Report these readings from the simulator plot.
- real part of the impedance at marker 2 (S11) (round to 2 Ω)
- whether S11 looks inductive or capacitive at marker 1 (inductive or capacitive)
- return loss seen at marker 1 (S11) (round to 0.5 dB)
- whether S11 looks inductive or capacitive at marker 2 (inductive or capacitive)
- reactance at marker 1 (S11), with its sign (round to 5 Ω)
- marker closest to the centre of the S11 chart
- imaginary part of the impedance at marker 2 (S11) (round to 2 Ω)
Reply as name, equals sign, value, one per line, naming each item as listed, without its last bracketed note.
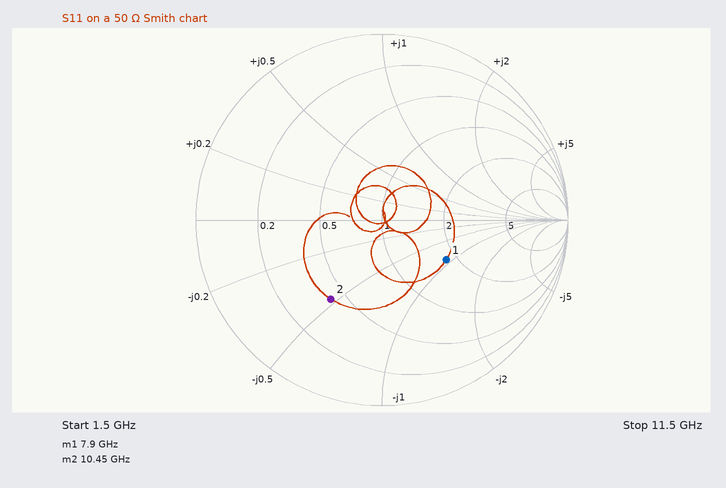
real part of the impedance at marker 2 (S11) = 20 Ω
whether S11 looks inductive or capacitive at marker 1 = capacitive
return loss seen at marker 1 (S11) = 8.0 dB
whether S11 looks inductive or capacitive at marker 2 = capacitive
reactance at marker 1 (S11), with its sign = -45 Ω
marker closest to the centre of the S11 chart = marker 1
imaginary part of the impedance at marker 2 (S11) = -24 Ω
